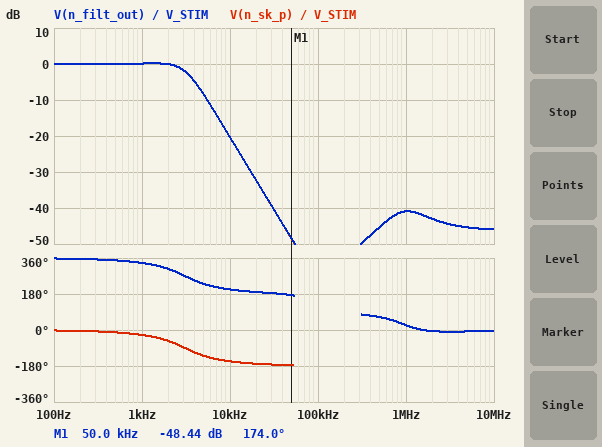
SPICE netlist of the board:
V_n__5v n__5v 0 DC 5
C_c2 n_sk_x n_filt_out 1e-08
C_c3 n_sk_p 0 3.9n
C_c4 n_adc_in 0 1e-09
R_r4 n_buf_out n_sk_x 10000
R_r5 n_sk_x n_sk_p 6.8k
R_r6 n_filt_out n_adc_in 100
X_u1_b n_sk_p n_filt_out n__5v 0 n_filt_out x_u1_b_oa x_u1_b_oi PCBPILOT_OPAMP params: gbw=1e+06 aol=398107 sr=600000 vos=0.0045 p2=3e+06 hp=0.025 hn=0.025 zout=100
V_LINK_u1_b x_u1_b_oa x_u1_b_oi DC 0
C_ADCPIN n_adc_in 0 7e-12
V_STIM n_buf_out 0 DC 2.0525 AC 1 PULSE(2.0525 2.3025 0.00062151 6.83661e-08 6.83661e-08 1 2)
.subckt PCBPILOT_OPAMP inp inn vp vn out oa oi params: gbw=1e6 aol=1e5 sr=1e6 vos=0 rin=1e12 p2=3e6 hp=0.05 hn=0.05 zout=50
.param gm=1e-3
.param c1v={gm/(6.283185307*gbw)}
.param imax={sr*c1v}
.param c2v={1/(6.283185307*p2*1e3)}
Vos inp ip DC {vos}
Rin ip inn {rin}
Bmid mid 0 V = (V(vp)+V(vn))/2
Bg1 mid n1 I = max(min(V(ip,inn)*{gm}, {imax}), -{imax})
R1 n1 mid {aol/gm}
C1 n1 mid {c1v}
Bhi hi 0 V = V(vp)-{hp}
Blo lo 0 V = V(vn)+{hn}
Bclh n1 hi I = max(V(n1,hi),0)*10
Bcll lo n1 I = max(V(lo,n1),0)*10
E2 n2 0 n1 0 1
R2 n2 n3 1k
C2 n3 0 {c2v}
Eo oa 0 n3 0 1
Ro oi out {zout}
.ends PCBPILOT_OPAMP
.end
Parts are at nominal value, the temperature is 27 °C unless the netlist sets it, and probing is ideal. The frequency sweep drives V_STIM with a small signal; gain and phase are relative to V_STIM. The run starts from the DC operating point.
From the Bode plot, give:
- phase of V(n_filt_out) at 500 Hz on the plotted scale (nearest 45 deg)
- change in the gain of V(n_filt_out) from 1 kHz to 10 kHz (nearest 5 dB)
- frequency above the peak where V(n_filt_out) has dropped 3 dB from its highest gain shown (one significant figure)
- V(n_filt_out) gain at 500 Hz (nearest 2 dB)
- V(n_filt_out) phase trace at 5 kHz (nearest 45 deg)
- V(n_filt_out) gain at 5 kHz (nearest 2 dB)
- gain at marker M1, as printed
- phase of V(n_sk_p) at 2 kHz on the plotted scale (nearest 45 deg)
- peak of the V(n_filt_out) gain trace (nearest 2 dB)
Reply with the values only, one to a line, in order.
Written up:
360 deg
-20 dB
3 kHz
0 dB
225 deg
-8 dB
-48.44 dB
-45 deg
0 dB
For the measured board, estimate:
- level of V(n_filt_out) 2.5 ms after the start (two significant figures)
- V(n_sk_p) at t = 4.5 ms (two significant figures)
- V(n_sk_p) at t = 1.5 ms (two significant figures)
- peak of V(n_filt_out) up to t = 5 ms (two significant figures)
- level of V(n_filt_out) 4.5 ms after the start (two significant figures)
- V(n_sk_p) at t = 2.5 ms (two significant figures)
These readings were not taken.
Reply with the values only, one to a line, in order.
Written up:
2.3 V
2.3 V
2.3 V
2.3 V
2.3 V
2.3 V
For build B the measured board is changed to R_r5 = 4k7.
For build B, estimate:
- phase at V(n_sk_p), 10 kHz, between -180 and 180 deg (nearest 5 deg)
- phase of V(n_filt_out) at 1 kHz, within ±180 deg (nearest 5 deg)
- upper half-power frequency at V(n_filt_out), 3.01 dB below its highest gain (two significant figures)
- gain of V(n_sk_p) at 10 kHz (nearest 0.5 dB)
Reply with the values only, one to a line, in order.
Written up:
-150 deg
-20 deg
3.9 kHz
-17.0 dB
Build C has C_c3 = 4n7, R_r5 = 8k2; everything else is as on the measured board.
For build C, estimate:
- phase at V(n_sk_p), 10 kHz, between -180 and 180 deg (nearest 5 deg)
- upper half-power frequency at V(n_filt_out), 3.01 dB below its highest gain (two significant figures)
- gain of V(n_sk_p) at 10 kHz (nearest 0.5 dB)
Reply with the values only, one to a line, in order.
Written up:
-160 deg
2.6 kHz
-23.5 dB
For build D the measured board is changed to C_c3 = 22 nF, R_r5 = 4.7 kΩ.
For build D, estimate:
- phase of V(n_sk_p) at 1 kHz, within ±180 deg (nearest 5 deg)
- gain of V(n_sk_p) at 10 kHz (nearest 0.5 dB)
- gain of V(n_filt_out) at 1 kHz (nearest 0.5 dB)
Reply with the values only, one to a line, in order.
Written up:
-75 deg
-33.0 dB
-6.5 dB
